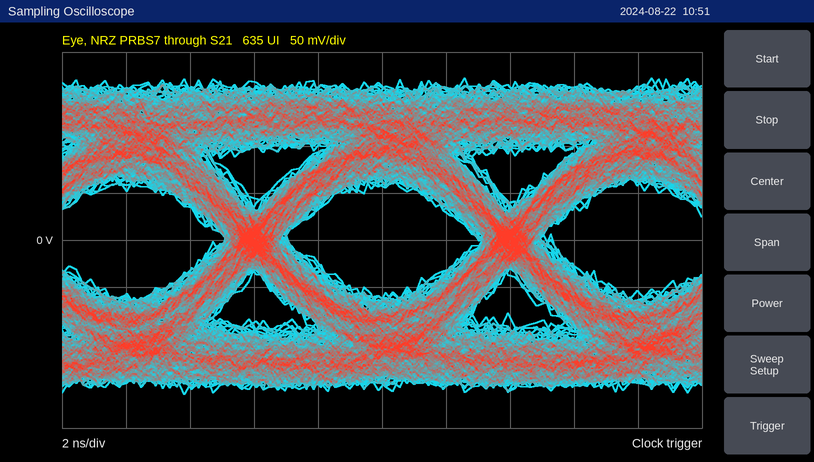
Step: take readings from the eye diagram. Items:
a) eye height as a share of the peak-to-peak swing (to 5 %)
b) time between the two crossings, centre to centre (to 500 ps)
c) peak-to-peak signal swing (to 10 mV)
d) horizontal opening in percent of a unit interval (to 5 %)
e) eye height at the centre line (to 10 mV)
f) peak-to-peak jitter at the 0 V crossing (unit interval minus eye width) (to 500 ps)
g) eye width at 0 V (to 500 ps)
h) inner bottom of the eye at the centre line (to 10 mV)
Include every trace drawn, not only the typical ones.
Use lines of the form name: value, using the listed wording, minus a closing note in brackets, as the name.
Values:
eye height as a share of the peak-to-peak swing: 35 %
time between the two crossings, centre to centre: 8.0 ns
peak-to-peak signal swing: 340 mV
horizontal opening in percent of a unit interval: 75 %
eye height at the centre line: 120 mV
peak-to-peak jitter at the 0 V crossing (unit interval minus eye width): 2.0 ns
eye width at 0 V: 6.0 ns
inner bottom of the eye at the centre line: -60 mV
